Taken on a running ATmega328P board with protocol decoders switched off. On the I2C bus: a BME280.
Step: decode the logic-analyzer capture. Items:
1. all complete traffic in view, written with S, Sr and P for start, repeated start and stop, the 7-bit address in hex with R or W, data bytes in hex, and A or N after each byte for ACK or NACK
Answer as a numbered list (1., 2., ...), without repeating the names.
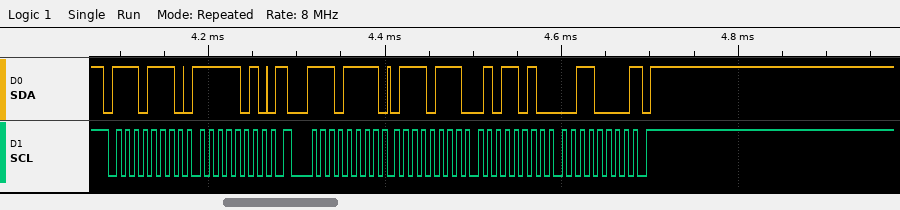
1. S 77W A FA A Sr 77R A 77 A 5A A 30 N P
